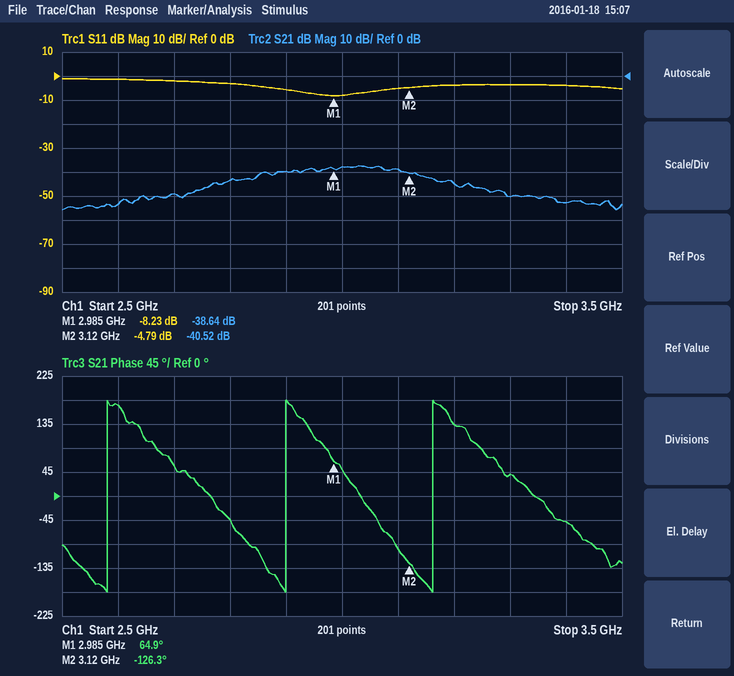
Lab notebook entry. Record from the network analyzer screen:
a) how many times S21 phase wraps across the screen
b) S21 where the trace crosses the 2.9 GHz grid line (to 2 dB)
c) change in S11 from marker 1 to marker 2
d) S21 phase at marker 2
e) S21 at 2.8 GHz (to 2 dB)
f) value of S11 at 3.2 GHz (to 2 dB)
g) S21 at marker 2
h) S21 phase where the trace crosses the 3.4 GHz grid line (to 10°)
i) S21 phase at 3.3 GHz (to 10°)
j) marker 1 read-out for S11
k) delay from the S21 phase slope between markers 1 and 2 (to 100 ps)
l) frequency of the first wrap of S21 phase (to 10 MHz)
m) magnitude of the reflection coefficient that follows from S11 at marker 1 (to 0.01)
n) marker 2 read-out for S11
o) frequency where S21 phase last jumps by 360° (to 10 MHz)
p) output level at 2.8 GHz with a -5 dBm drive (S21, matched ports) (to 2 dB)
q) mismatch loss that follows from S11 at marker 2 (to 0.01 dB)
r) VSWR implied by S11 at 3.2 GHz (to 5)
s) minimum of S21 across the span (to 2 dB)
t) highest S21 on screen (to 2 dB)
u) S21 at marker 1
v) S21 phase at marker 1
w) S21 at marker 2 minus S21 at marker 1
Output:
3
-40 dB
3.44 dB
-126.3°
-44 dB
-4 dB
-40.52 dB
-50°
40°
-8.23 dB
3.9 ns
2.58 GHz
0.39
-4.79 dB
3.16 GHz
-48 dBm
1.75 dB
5
-56 dB
-38 dB
-38.64 dB
64.9°
-1.88 dB
